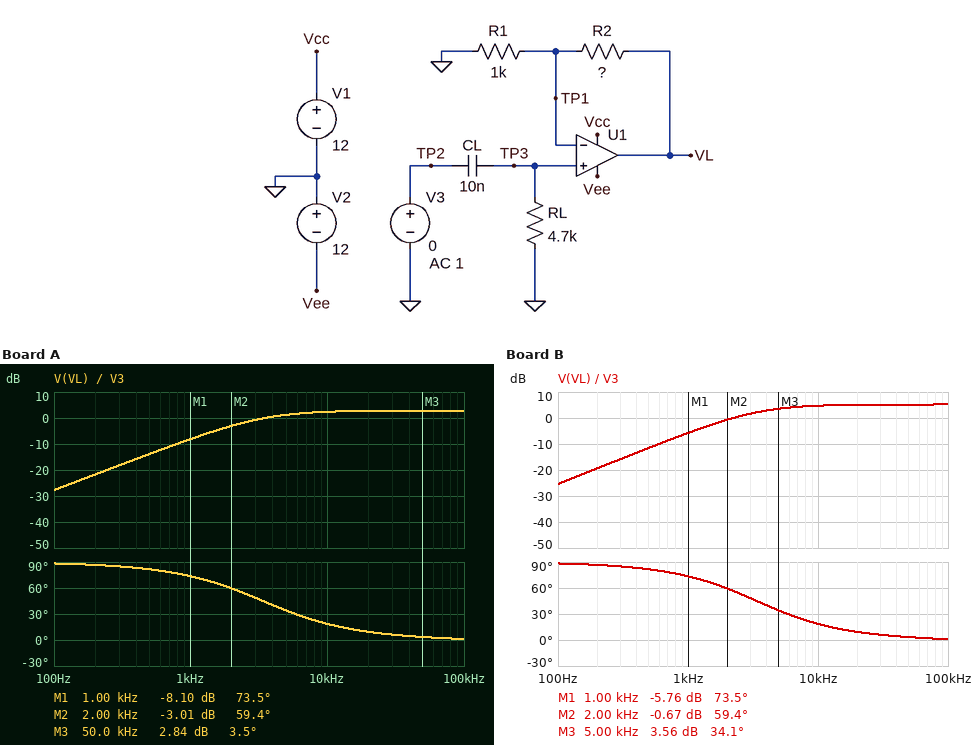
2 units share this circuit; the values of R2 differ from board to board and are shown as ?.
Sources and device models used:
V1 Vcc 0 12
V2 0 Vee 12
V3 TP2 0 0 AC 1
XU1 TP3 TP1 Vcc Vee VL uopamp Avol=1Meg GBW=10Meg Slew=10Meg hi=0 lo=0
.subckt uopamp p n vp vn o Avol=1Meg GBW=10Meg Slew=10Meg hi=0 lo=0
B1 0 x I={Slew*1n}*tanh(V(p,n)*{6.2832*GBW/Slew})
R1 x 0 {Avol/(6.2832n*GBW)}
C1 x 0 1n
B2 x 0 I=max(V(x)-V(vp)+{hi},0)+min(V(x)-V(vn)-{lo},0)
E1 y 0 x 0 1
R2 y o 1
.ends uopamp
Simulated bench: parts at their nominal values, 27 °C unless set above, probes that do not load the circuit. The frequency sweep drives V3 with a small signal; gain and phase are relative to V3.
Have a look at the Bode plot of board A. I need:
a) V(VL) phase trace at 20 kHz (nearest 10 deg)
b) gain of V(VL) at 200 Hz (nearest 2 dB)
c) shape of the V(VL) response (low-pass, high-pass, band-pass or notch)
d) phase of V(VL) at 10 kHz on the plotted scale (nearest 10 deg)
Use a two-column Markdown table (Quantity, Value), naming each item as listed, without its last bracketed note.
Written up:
| Quantity | Value |
|---|---|
| V(VL) phase trace at 20 kHz | 10 deg |
| gain of V(VL) at 200 Hz | -22 dB |
| shape of the V(VL) response | high-pass |
| phase of V(VL) at 10 kHz on the plotted scale | 20 deg |
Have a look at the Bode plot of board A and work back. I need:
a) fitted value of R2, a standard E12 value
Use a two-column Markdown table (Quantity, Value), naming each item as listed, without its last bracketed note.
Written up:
| Quantity | Value |
|---|---|
| fitted value of R2, a standard E12 value | 390 Ω |
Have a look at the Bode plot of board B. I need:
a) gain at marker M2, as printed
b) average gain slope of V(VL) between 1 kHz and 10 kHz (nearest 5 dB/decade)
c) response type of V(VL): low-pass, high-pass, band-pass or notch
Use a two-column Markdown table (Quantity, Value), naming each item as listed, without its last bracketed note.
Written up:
| Quantity | Value |
|---|---|
| gain at marker M2, as printed | -0.67 dB |
| average gain slope of V(VL) between 1 kHz and 10 kHz | 10 dB/decade |
| response type of V(VL): low-pass, high-pass, band-pass or notch | high-pass |
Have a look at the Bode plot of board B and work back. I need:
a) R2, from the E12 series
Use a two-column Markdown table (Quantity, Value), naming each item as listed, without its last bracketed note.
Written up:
| Quantity | Value |
|---|---|
| R2, from the E12 series | 820 Ω |
